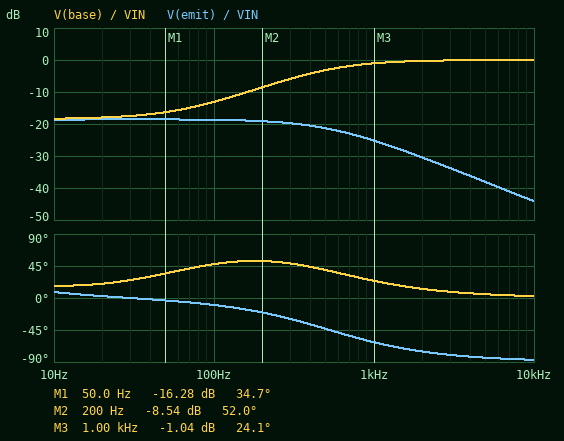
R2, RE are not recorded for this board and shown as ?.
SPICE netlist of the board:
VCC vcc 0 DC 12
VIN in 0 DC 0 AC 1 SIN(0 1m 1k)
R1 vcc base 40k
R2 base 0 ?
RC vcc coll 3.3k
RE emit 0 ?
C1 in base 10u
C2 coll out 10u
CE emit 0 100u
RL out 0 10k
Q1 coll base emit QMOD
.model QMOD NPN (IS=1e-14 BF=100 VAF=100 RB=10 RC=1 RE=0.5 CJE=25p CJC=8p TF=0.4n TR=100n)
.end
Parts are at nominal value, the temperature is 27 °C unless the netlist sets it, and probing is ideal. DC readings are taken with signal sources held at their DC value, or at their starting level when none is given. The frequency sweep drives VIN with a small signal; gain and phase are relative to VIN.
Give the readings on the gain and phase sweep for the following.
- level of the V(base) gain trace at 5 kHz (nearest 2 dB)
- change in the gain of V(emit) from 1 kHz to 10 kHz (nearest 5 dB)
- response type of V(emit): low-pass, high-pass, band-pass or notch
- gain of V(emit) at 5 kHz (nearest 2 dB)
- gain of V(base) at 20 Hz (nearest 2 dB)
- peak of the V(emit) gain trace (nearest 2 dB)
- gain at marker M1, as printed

0 dB
-20 dB
low-pass
-38 dB
-18 dB
-18 dB
-16.28 dB
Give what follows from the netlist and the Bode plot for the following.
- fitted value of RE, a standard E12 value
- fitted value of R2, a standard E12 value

1.5 kΩ
33 kΩ
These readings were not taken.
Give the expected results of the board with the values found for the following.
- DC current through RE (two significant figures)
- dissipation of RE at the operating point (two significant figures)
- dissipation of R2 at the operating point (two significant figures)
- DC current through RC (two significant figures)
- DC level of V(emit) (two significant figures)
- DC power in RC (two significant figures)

2.5 mA
9.5 mW
600 µW
2.5 mA
3.8 V
20 mW
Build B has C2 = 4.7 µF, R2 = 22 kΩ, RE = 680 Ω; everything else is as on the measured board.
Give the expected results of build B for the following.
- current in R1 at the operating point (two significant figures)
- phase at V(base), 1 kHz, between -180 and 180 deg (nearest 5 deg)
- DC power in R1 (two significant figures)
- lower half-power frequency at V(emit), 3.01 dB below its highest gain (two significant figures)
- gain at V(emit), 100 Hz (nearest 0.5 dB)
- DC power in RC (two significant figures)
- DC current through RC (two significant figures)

230 µA
30 deg
2.1 mW
2.8 Hz
-20.0 dB
29 mW
3.0 mA
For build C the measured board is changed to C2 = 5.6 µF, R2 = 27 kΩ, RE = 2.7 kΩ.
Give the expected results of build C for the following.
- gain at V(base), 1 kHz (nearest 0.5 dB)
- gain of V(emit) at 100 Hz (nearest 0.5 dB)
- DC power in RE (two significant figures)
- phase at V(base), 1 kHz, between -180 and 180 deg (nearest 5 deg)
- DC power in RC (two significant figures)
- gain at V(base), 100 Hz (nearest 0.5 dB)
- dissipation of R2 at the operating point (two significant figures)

0 dB
-4.0 dB
5.8 mW
0 deg
6.9 mW
-0.5 dB
790 µW
